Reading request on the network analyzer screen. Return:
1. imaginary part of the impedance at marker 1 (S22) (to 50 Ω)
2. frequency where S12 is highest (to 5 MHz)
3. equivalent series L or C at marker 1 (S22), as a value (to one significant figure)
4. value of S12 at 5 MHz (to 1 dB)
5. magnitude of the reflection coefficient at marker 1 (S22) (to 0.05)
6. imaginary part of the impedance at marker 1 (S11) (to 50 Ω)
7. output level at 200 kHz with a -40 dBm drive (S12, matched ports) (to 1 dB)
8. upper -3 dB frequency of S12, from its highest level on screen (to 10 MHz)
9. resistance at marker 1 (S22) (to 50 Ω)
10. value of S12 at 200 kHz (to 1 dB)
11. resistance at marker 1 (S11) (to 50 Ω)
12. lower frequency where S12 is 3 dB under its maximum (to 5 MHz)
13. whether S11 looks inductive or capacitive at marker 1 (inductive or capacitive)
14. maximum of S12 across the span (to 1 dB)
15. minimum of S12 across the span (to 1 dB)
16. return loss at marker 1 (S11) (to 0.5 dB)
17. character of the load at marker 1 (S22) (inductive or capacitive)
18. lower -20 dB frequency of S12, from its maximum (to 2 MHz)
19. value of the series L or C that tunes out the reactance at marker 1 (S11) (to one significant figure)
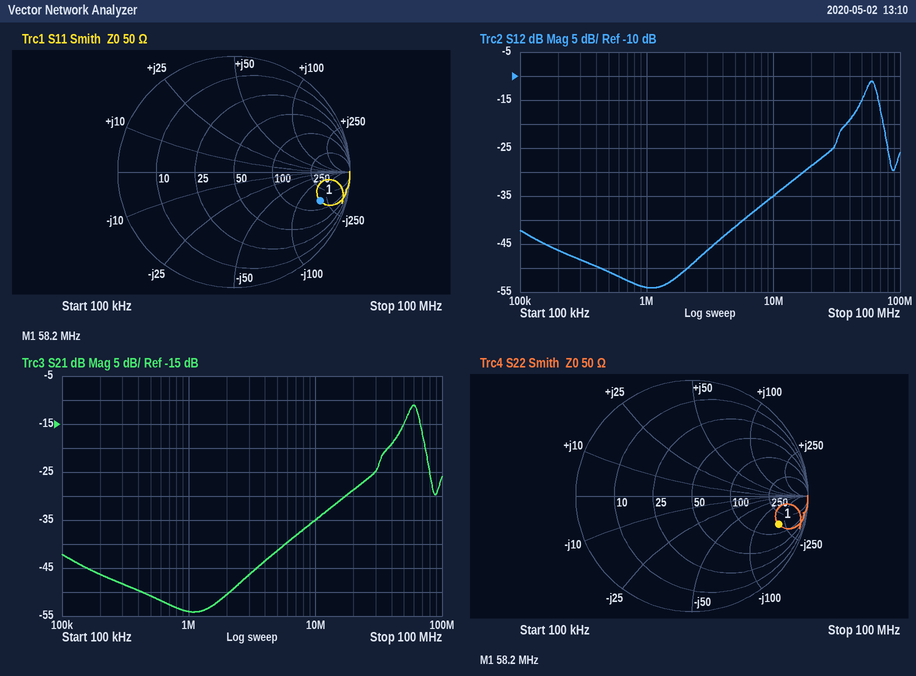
-200 Ω
60 MHz
10 pF
-41 dB
0.80
-200 Ω
-86 dBm
70 MHz
150 Ω
-46 dB
150 Ω
50 MHz
capacitive
-11 dB
-54 dB
2.0 dB
capacitive
16 MHz
500 nH
